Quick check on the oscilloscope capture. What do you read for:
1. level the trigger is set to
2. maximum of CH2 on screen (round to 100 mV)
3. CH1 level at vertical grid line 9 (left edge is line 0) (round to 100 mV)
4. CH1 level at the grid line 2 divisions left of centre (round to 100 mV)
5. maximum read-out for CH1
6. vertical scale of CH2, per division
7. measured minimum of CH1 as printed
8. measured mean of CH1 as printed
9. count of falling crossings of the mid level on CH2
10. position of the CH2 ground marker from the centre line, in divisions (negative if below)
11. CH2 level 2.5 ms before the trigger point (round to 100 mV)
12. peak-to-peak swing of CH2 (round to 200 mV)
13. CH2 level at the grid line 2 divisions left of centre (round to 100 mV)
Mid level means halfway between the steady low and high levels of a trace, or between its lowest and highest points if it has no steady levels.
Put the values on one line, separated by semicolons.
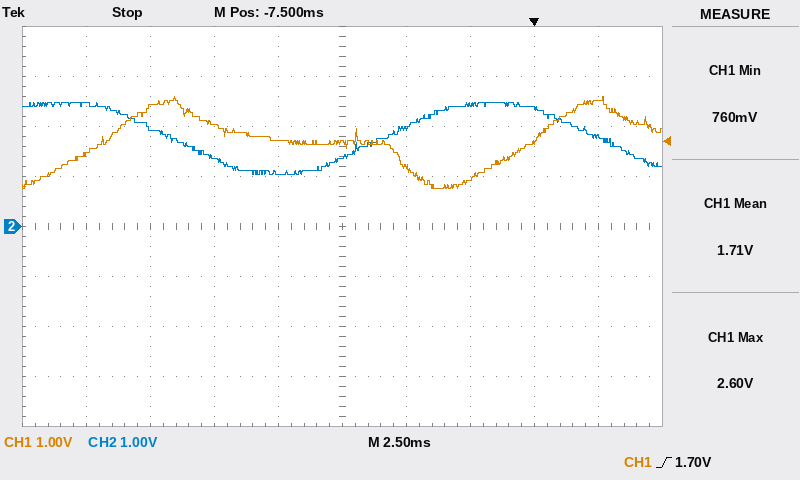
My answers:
1.70 V; 2.5 V; 2.5 V; 2.0 V; 2.60 V; 1 V; 760 mV; 1.71 V; 2; 0.0 div; 2.4 V; 1.4 V; 1.4 V
